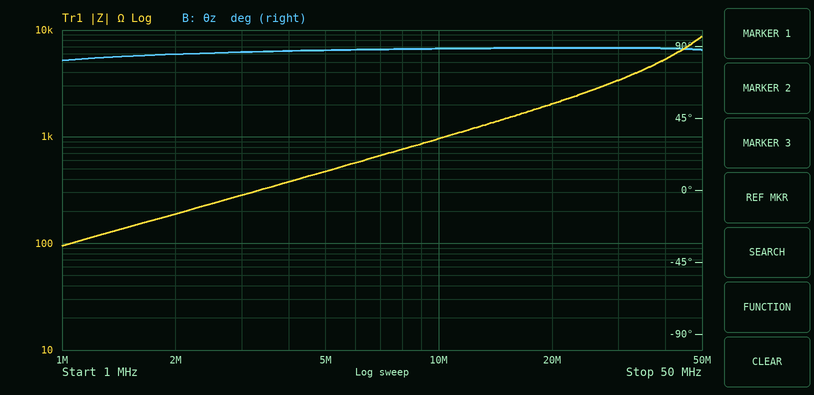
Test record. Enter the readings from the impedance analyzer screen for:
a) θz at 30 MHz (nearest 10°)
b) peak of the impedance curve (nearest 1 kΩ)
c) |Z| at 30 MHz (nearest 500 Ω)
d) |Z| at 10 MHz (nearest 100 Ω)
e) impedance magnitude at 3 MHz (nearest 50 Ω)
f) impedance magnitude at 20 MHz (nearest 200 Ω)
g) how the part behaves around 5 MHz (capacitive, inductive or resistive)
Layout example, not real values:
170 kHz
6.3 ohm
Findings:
90°
9 kΩ
3.5 kΩ
1.0 kΩ
300 Ω
2.0 kΩ
inductive
